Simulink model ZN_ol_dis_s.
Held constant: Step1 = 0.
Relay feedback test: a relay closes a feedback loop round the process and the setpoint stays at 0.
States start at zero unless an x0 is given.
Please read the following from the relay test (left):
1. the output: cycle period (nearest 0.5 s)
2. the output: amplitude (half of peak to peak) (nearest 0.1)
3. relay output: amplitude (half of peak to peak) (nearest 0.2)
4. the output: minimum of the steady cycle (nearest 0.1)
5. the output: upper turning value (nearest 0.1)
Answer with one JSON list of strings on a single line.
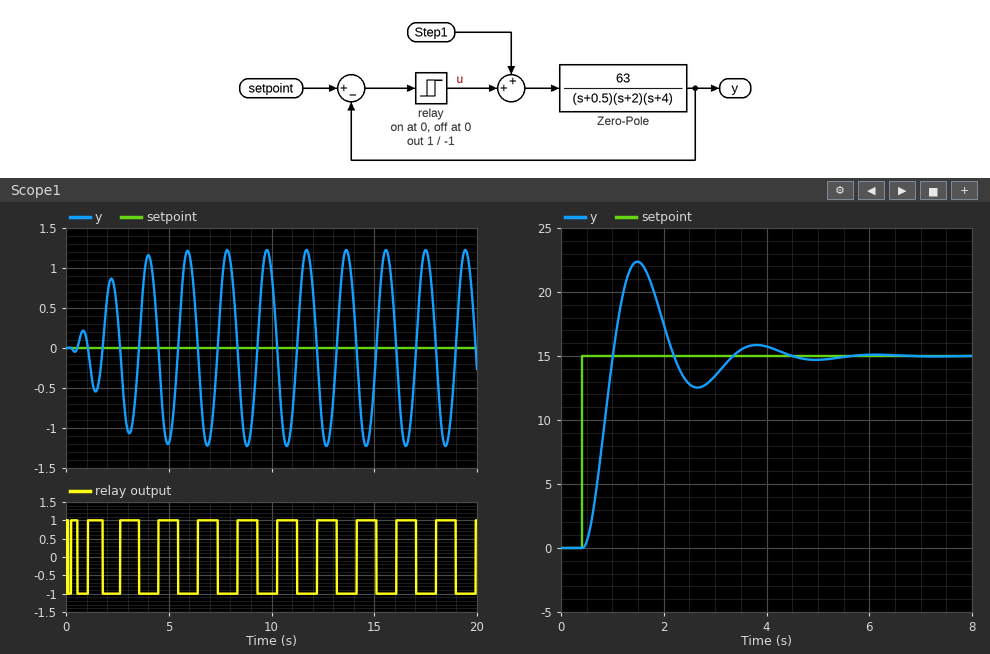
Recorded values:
["2.0 s", "1.2", "1.0", "-1.2", "1.2"]
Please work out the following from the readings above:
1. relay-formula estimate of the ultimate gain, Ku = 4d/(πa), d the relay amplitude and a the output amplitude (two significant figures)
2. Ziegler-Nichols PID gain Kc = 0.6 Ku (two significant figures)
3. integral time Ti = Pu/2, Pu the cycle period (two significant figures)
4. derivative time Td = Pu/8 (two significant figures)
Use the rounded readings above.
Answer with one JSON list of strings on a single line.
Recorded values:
["1.1", "0.66", "1.0 s", "0.25 s"]
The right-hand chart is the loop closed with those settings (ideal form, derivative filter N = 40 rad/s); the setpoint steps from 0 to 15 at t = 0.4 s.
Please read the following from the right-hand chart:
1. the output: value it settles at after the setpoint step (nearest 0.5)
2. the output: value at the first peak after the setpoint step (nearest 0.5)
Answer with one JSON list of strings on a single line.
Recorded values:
["15.0", "22.5"]
